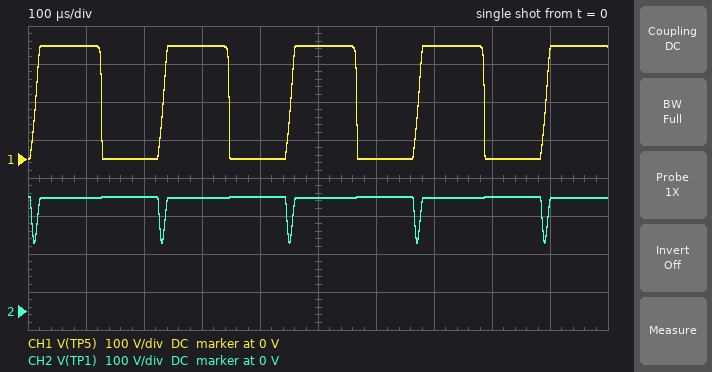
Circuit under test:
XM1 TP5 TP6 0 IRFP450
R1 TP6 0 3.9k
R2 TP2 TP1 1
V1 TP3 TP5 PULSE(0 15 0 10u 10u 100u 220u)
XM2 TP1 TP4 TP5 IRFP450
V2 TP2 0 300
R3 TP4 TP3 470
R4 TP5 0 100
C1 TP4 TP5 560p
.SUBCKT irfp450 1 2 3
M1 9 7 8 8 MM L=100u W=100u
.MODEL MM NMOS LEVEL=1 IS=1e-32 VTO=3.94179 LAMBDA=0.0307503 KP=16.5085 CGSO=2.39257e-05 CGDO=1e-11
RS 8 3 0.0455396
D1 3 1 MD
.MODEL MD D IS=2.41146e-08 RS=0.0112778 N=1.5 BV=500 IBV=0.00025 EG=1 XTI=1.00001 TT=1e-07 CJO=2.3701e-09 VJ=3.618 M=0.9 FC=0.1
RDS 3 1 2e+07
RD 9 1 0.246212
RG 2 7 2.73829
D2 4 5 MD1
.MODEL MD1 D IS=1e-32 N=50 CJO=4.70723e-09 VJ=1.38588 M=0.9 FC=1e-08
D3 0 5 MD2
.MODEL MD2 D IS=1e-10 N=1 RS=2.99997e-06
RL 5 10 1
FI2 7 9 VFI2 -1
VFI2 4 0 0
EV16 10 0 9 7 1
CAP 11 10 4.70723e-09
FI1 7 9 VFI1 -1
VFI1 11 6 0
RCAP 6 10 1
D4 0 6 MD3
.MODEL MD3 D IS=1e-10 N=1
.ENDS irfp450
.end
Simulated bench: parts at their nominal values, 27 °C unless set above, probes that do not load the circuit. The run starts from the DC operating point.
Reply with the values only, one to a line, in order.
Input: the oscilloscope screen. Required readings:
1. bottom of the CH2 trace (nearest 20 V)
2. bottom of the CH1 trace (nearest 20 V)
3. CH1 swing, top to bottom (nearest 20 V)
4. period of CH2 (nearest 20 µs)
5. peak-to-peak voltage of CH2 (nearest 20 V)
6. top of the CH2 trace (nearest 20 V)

180 V
0 V
300 V
220 µs
120 V
300 V
